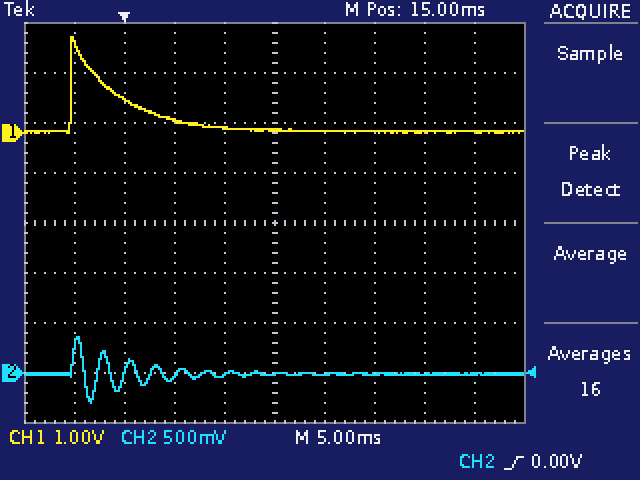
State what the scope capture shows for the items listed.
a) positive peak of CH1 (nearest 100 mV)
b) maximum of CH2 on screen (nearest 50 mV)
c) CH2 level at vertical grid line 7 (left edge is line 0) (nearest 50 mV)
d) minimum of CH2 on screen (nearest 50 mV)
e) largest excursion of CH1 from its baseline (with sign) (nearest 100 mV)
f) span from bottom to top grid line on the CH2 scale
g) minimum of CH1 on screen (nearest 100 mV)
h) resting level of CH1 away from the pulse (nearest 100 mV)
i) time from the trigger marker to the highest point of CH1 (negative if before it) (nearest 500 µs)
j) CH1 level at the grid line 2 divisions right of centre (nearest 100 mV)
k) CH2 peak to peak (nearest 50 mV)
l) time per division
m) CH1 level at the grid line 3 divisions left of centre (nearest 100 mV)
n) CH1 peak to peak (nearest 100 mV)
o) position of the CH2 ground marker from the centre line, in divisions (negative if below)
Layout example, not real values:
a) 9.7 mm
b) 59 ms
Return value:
a) 1.9 V
b) 350 mV
c) 0 mV
d) -300 mV
e) +1.9 V
f) 4 V
g) 0.0 V
h) 0.0 V
i) -5.0 ms
j) 0.0 V
k) 650 mV
l) 5 ms
m) 700 mV
n) 1.9 V
o) -3.0 div
